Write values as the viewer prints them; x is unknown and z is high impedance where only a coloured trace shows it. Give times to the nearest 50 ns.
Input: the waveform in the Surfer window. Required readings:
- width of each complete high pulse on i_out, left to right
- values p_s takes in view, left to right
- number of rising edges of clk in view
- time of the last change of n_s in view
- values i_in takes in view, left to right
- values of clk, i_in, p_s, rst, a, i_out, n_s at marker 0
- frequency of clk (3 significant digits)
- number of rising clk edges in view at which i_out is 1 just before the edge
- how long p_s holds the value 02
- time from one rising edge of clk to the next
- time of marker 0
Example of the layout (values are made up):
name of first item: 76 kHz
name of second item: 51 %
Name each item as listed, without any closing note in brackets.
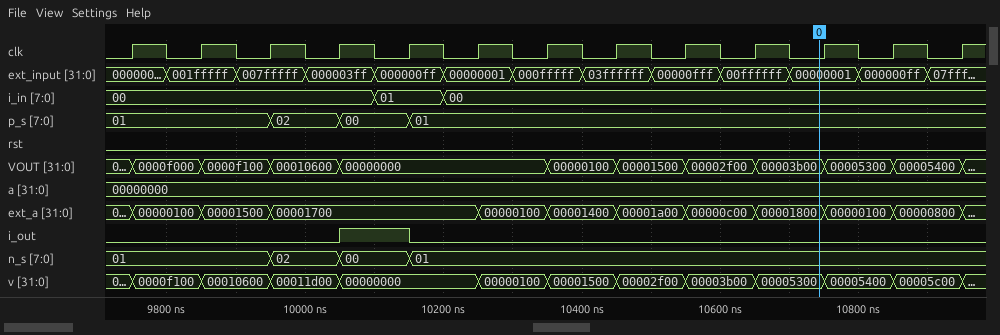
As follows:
width of each complete high pulse on i_out, left to right: 100 ns
values p_s takes in view, left to right: 01, 02, 00, 01
number of rising edges of clk in view: 13
time of the last change of n_s in view: 10150 ns
values i_in takes in view, left to right: 00, 01, 00
values of clk, i_in, p_s, rst, a, i_out, n_s at marker 0: clk=0, i_in=00, p_s=01, rst=0, a=00000000, i_out=0, n_s=01
frequency of clk: 10.0 MHz
number of rising clk edges in view at which i_out is 1 just before the edge: 1
how long p_s holds the value 02: 100 ns
time from one rising edge of clk to the next: 100 ns
time of marker 0: 10750 ns
